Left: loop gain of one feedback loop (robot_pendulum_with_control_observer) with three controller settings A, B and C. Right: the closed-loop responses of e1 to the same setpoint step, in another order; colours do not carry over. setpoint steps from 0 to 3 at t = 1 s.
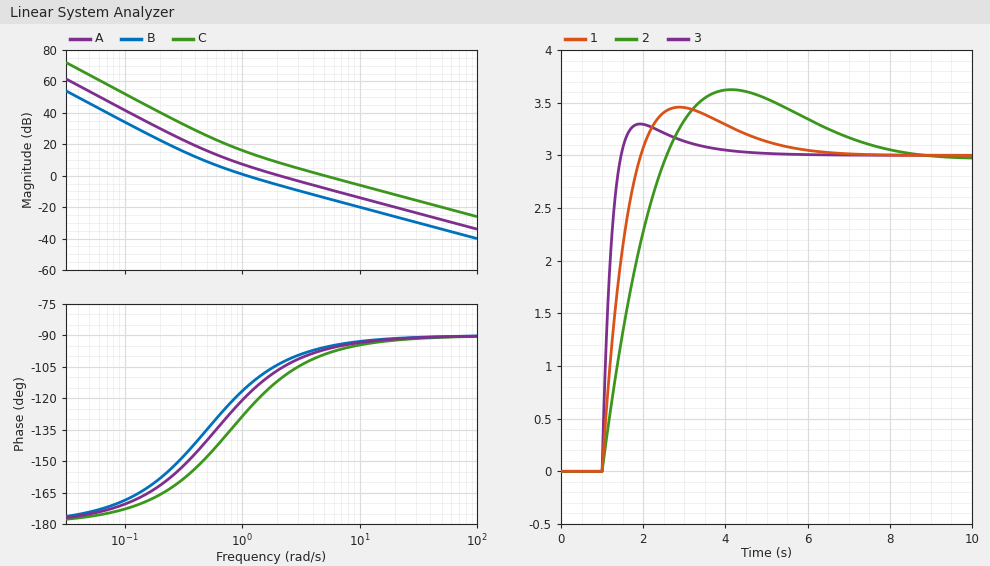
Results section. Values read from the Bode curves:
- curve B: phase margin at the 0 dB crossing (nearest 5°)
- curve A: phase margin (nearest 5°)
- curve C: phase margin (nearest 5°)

65°
75°
80°
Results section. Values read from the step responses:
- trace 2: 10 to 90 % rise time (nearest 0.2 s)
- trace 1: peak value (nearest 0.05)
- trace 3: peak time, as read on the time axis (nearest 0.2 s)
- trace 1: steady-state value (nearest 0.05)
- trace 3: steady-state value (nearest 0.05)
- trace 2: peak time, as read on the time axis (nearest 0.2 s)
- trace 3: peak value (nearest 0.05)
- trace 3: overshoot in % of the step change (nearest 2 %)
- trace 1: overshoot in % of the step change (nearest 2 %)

1.2 s
3.45
2.0 s
3.00
3.00
4.2 s
3.30
10 %
16 %
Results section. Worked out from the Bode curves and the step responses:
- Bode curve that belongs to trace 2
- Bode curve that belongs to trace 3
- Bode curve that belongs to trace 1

B
C
A
